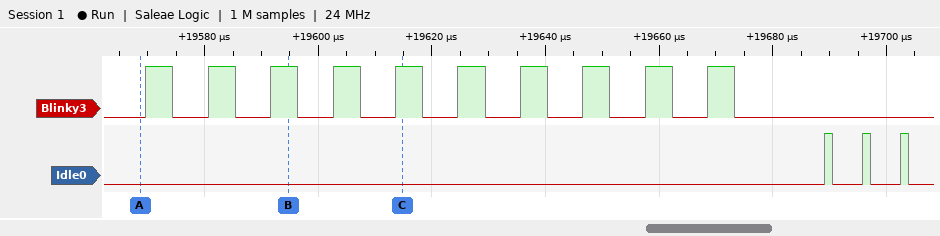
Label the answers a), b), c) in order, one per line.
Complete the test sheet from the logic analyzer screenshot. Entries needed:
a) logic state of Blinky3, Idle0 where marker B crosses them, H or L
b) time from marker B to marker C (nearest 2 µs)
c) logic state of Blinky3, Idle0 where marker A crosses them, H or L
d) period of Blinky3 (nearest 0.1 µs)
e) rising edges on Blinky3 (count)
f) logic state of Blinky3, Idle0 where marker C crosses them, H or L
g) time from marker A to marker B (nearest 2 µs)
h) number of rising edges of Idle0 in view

a) Blinky3=H, Idle0=L
b) 20 µs
c) Blinky3=L, Idle0=L
d) 11 µs
e) 10
f) Blinky3=H, Idle0=L
g) 26 µs
h) 3
